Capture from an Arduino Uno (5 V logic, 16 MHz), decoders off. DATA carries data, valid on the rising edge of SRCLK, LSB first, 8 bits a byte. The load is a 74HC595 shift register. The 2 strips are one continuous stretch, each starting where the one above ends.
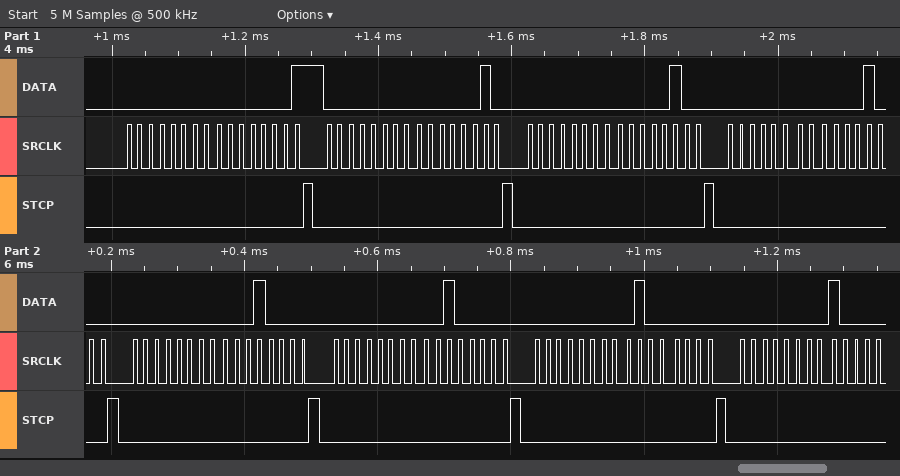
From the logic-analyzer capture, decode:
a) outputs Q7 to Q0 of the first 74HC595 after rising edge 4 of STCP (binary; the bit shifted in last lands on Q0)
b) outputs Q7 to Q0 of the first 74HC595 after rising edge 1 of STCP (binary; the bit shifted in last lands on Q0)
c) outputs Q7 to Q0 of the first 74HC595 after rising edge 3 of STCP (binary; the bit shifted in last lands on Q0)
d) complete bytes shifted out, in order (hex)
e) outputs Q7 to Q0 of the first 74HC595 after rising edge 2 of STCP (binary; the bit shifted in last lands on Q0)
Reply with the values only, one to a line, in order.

00001000
00000001
00000100
00 80 00 40 00 20 00 10 00 08 00 04 00 02 00
00000010
